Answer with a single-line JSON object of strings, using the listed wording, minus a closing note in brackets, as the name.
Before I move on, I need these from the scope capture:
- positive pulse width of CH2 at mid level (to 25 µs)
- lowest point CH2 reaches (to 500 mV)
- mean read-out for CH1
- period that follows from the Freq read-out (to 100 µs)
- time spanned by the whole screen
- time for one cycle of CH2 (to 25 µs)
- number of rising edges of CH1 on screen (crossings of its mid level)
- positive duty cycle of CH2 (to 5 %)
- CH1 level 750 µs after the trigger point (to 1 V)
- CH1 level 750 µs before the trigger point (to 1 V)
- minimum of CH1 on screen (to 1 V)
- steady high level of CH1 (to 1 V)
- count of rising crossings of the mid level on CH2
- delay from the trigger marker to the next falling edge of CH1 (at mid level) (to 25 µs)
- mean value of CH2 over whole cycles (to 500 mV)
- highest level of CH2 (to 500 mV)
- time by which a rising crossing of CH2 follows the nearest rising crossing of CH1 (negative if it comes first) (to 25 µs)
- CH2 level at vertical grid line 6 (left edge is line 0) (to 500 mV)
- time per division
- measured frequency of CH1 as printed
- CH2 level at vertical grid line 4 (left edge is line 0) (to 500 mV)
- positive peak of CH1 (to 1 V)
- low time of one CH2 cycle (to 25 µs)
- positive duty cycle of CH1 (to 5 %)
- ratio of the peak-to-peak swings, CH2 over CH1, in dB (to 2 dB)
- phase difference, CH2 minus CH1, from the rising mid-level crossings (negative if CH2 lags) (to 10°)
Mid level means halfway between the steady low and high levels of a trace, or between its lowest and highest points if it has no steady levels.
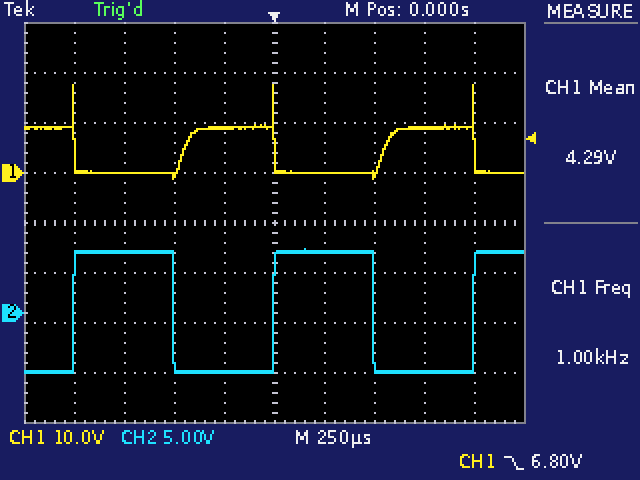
{"positive pulse width of CH2 at mid level": "500 µs", "lowest point CH2 reaches": "-6.0 V", "mean read-out for CH1": "4.29 V", "period that follows from the Freq read-out": "1.0 ms", "time spanned by the whole screen": "2.5 ms", "time for one cycle of CH2": "1.000 ms", "number of rising edges of CH1 on screen": "2", "positive duty cycle of CH2": "50 %", "CH1 level 750 µs after the trigger point": "9 V", "CH1 level 750 µs before the trigger point": "0 V", "minimum of CH1 on screen": "-1 V", "steady high level of CH1": "9 V", "count of rising crossings of the mid level on CH2": "3", "delay from the trigger marker to the next falling edge of CH1 (at mid level)": "1.000 ms", "mean value of CH2 over whole cycles": "0.0 V", "highest level of CH2": "6.5 V", "time by which a rising crossing of CH2 follows the nearest rising crossing of CH1 (negative if it comes first)": "+450 µs", "CH2 level at vertical grid line 6 (left edge is line 0)": "6.0 V", "time per division": "250 µs", "measured frequency of CH1 as printed": "1.00 kHz", "CH2 level at vertical grid line 4 (left edge is line 0)": "-6.0 V", "positive peak of CH1": "18 V", "low time of one CH2 cycle": "500 µs", "positive duty cycle of CH1": "45 %", "ratio of the peak-to-peak swings, CH2 over CH1, in dB": "-4 dB", "phase difference, CH2 minus CH1, from the rising mid-level crossings (negative if CH2 lags)": "-160°"}
